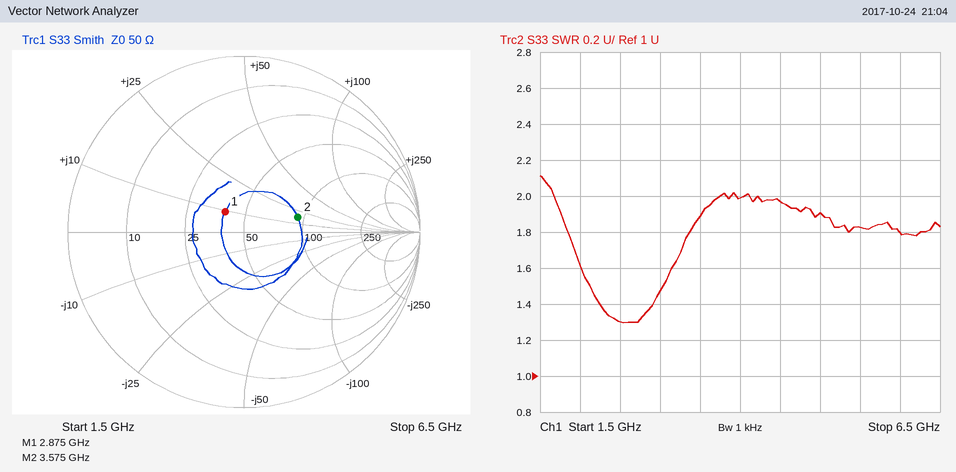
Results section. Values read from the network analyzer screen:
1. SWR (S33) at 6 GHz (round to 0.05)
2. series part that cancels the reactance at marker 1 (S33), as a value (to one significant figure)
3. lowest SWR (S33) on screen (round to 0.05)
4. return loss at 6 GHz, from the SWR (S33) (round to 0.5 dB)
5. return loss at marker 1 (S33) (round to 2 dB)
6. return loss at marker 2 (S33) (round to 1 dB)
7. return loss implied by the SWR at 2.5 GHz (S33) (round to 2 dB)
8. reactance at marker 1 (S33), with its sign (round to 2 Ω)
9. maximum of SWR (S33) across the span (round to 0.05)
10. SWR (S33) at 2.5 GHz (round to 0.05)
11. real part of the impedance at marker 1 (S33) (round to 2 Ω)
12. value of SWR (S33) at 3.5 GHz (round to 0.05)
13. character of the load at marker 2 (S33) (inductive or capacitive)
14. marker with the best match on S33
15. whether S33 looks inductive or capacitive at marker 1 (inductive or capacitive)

1.80
6 pF
1.30
11.0 dB
16 dB
10 dB
18 dB
+10 Ω
2.10
1.30
40 Ω
1.90
inductive
marker 1
inductive
